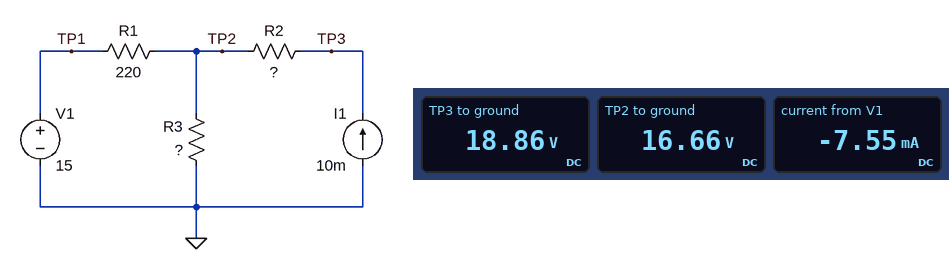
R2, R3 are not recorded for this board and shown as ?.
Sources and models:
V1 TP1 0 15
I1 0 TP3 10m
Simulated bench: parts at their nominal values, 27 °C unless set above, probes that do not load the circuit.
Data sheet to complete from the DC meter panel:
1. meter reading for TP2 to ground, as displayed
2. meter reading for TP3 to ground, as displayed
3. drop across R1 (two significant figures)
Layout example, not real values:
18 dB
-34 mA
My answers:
16.66 V
18.86 V
1.7 V
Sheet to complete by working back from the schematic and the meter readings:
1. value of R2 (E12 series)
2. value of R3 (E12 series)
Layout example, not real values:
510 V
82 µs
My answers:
220 Ω
6.8 kΩ
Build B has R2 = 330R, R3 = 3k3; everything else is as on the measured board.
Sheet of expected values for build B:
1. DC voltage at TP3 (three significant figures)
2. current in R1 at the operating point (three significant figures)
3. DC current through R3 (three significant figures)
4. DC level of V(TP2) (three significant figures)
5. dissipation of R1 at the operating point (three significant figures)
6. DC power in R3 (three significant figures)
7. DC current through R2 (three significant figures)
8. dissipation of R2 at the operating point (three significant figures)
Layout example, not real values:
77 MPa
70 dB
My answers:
19.4 V
5.11 mA
4.89 mA
16.1 V
5.75 mW
78.8 mW
10.0 mA
33.0 mW
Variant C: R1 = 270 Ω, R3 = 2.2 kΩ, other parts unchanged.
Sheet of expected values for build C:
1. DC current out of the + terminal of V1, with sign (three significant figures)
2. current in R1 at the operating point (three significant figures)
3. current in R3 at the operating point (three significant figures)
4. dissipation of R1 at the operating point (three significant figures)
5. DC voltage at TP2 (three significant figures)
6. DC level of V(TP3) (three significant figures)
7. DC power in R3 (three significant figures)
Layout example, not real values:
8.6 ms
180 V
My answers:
-2.83 mA
2.83 mA
7.17 mA
2.17 mW
15.8 V
18.0 V
113 mW
